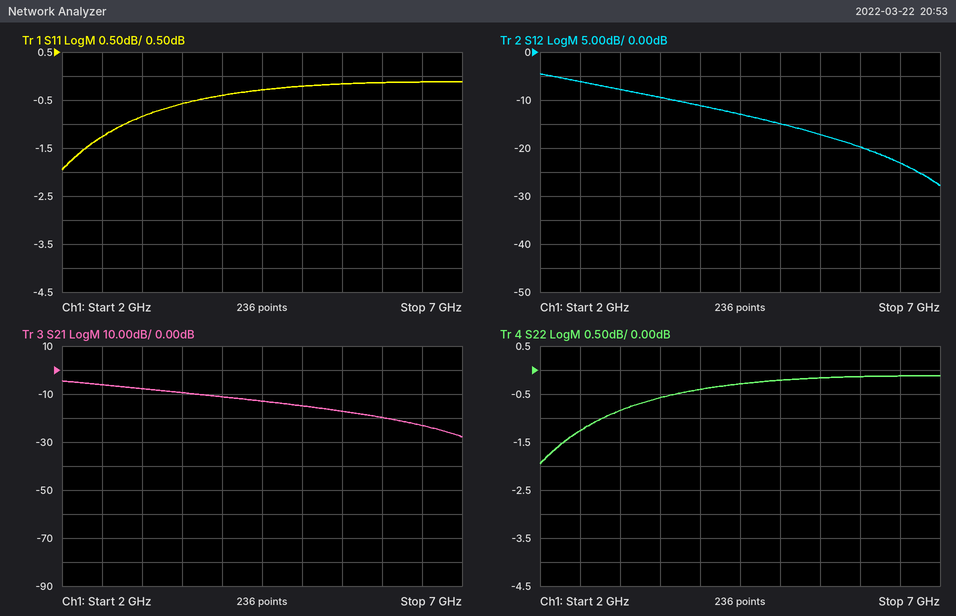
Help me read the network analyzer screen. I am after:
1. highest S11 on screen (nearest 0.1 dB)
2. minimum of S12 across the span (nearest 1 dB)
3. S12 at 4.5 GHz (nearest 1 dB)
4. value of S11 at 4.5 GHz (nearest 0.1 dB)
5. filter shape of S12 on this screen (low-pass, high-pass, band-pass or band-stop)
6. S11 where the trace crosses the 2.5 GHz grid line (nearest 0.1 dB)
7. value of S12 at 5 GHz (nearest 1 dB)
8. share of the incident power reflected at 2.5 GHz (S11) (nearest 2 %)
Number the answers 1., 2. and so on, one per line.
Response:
1. -0.1 dB
2. -28 dB
3. -13 dB
4. -0.3 dB
5. low-pass
6. -1.3 dB
7. -15 dB
8. 74 %
